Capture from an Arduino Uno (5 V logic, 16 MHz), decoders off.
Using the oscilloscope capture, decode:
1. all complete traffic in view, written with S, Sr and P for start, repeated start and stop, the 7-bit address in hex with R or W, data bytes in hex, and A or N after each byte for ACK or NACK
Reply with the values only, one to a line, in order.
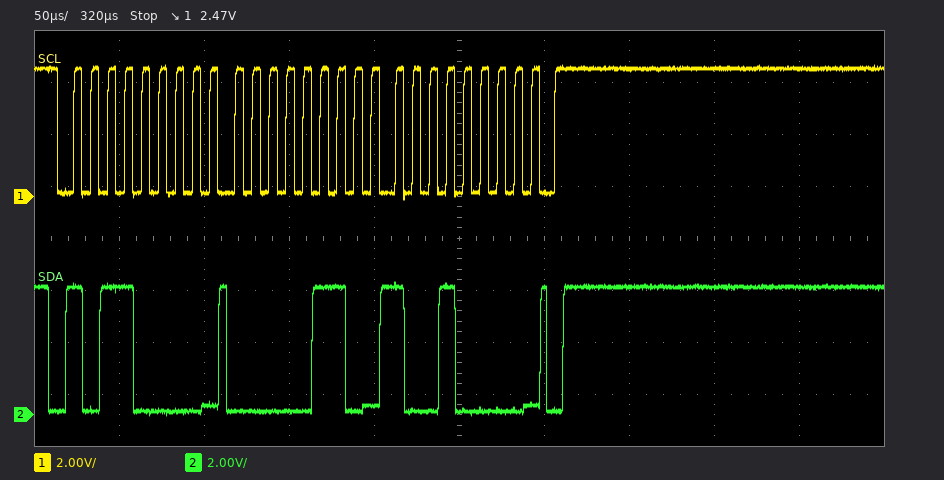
S 58W A 06 A 90 A P
